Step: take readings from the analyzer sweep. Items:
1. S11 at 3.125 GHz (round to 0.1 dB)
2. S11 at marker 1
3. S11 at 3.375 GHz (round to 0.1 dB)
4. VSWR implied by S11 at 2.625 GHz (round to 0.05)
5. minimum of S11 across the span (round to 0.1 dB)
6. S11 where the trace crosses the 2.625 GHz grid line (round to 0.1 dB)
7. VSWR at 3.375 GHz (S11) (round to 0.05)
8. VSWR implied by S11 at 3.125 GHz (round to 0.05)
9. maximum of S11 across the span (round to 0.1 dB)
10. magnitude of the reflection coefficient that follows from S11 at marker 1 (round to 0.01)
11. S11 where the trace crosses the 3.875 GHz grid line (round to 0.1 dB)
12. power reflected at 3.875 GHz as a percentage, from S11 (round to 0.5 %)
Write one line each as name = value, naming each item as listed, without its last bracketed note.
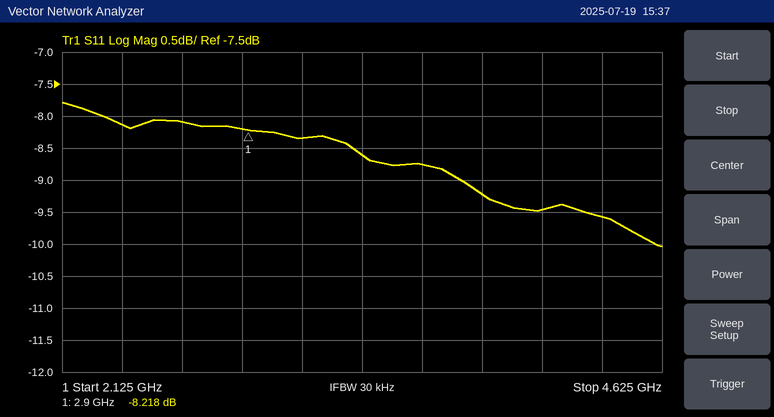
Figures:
S11 at 3.125 GHz = -8.3 dB
S11 at marker 1 = -8.218 dB
S11 at 3.375 GHz = -8.6 dB
VSWR implied by S11 at 2.625 GHz = 2.30
minimum of S11 across the span = -10.0 dB
S11 where the trace crosses the 2.625 GHz grid line = -8.1 dB
VSWR at 3.375 GHz (S11) = 2.20
VSWR implied by S11 at 3.125 GHz = 2.25
maximum of S11 across the span = -7.8 dB
magnitude of the reflection coefficient that follows from S11 at marker 1 = 0.39
S11 where the trace crosses the 3.875 GHz grid line = -9.2 dB
power reflected at 3.875 GHz as a percentage, from S11 = 12.0 %
